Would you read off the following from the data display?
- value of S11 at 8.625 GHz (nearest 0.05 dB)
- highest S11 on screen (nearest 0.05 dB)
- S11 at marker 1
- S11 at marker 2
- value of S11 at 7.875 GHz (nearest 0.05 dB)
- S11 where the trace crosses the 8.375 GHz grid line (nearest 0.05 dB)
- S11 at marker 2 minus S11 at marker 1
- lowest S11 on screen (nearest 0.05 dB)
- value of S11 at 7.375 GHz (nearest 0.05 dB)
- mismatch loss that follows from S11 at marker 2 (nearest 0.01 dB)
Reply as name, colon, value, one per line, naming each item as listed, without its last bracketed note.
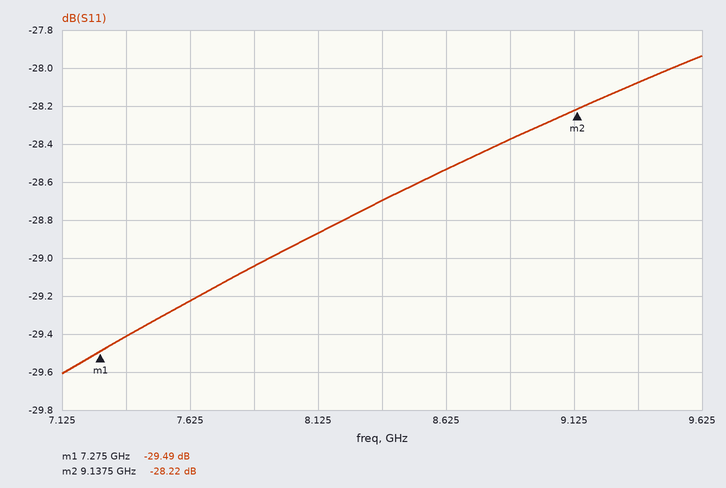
value of S11 at 8.625 GHz: -28.55 dB
highest S11 on screen: -27.95 dB
S11 at marker 1: -29.49 dB
S11 at marker 2: -28.22 dB
value of S11 at 7.875 GHz: -29.05 dB
S11 where the trace crosses the 8.375 GHz grid line: -28.70 dB
S11 at marker 2 minus S11 at marker 1: 1.27 dB
lowest S11 on screen: -29.60 dB
value of S11 at 7.375 GHz: -29.40 dB
mismatch loss that follows from S11 at marker 2: 0.01 dB
